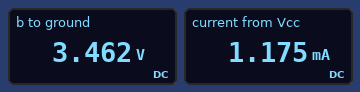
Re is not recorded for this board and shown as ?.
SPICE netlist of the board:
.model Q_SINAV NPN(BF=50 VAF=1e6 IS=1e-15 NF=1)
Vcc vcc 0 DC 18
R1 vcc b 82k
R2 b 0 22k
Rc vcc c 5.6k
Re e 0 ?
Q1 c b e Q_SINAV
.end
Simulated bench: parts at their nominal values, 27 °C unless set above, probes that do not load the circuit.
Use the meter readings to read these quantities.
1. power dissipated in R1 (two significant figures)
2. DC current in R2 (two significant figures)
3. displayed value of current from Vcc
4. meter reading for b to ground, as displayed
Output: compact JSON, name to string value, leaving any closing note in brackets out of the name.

{"power dissipated in R1": "2.6 mW", "DC current in R2": "160 µA", "displayed value of current from Vcc": "1.175 mA", "meter reading for b to ground, as displayed": "3.462 V"}
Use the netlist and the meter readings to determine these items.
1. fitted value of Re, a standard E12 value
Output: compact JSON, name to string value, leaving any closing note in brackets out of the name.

{"fitted value of Re, a standard E12 value": "2.7 kΩ"}
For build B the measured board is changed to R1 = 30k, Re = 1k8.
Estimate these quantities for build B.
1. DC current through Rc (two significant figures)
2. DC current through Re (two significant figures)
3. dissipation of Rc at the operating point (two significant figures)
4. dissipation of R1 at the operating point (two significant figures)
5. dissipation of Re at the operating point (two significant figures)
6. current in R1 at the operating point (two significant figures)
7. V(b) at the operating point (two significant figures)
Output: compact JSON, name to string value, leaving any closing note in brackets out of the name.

{"DC current through Rc": "2.4 mA", "DC current through Re": "2.6 mA", "dissipation of Rc at the operating point": "32 mW", "dissipation of R1 at the operating point": "5.3 mW", "dissipation of Re at the operating point": "12 mW", "current in R1 at the operating point": "420 µA", "V(b) at the operating point": "5.3 V"}
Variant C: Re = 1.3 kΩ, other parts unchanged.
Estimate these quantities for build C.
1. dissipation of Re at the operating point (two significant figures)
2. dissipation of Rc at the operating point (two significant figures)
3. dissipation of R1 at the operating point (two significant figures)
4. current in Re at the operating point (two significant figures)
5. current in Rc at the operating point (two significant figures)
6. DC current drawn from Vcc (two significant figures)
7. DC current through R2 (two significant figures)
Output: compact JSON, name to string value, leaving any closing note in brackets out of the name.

{"dissipation of Re at the operating point": "4.6 mW", "dissipation of Rc at the operating point": "19 mW", "dissipation of R1 at the operating point": "2.7 mW", "current in Re at the operating point": "1.9 mA", "current in Rc at the operating point": "1.8 mA", "DC current drawn from Vcc": "2.0 mA", "DC current through R2": "140 µA"}
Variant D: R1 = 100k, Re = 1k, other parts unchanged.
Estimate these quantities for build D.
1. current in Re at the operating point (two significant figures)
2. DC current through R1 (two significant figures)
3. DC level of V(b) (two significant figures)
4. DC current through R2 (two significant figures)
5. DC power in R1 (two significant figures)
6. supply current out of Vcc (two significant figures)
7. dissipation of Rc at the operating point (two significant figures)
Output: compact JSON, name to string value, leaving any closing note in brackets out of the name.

{"current in Re at the operating point": "1.9 mA", "DC current through R1": "150 µA", "DC level of V(b)": "2.6 V", "DC current through R2": "120 µA", "DC power in R1": "2.4 mW", "supply current out of Vcc": "2.0 mA", "dissipation of Rc at the operating point": "19 mW"}
